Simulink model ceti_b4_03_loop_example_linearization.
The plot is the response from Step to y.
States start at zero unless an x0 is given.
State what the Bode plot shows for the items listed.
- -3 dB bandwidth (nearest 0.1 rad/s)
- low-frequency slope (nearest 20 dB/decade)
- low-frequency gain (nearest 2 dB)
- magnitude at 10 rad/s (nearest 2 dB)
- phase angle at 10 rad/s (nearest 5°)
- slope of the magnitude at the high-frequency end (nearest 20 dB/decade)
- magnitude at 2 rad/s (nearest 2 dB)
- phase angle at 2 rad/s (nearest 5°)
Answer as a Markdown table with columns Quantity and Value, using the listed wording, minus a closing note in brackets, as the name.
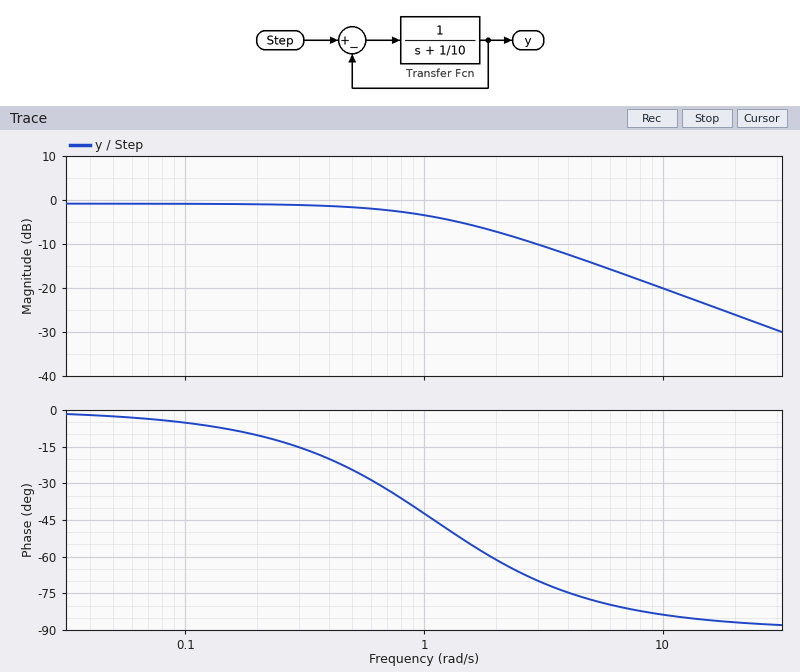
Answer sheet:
| Quantity | Value |
|---|---|
| -3 dB bandwidth | 1.1 rad/s |
| low-frequency slope | 0 dB/decade |
| low-frequency gain | 0 dB |
| magnitude at 10 rad/s | -20 dB |
| phase angle at 10 rad/s | -85° |
| slope of the magnitude at the high-frequency end | -20 dB/decade |
| magnitude at 2 rad/s | -8 dB |
| phase angle at 2 rad/s | -60° |
